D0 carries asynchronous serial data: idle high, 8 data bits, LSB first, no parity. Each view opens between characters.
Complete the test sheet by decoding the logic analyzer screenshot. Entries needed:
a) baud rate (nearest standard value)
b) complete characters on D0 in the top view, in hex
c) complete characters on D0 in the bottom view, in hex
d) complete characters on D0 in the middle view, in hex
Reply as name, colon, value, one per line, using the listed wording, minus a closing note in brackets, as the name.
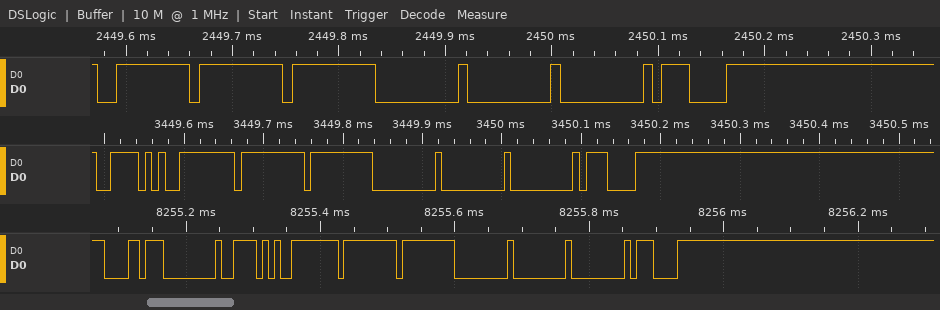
baud rate: 115200 baud
complete characters on D0 in the top view, in hex: FE, FF, FF, 00, 00, 00, 87
complete characters on D0 in the bottom view, in hex: D8, 00, 5E, FE, FF, FF, 00, 00, 00, 87
complete characters on D0 in the middle view, in hex: 5E, FE, FF, FF, 00, 00, 00, 87
